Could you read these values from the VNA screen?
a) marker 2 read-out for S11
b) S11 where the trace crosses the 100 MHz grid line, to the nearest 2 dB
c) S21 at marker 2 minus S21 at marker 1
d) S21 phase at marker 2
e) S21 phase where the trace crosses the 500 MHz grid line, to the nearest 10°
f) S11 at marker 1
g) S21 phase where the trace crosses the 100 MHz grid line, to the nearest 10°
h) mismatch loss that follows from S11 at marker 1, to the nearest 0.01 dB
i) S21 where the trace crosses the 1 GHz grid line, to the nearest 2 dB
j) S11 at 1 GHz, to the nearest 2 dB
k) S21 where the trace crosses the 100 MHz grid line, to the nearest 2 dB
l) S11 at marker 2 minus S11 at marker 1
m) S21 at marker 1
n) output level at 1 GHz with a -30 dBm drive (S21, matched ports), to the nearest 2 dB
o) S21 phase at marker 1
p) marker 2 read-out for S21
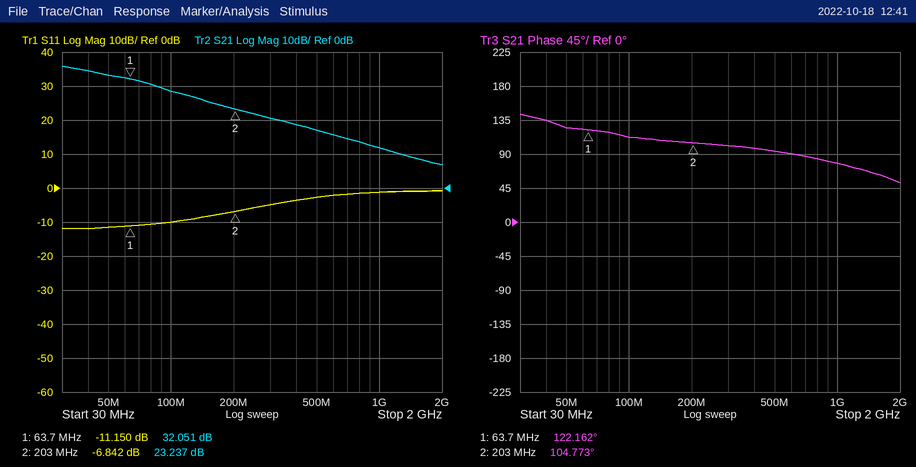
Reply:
-6.842 dB
-10 dB
-8.814 dB
104.773°
90°
-11.150 dB
110°
0.35 dB
12 dB
-2 dB
28 dB
4.308 dB
32.051 dB
-18 dBm
122.162°
23.237 dB
